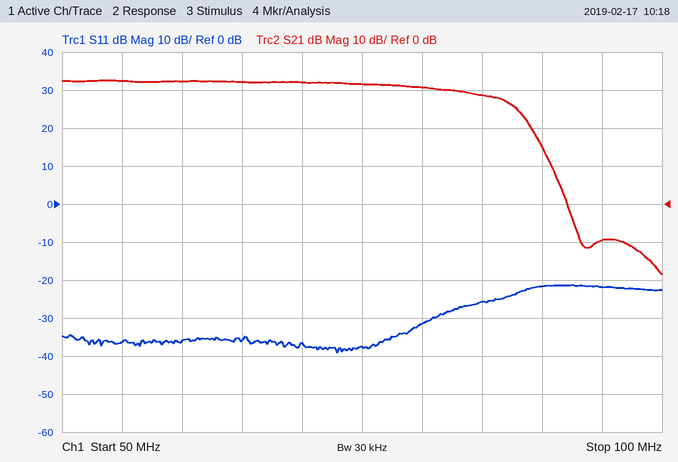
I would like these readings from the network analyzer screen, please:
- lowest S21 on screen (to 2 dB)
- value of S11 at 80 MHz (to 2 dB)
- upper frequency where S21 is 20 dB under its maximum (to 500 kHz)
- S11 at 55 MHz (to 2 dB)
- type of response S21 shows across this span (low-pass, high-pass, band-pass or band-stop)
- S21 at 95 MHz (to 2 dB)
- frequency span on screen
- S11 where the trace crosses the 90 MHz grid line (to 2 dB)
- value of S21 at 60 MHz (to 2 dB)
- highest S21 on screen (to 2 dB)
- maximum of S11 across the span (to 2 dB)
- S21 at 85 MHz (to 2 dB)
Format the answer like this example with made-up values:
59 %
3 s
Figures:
-18 dB
-32 dB
90.5 MHz
-36 dB
low-pass
-10 dB
50 MHz
-22 dB
32 dB
32 dB
-22 dB
28 dB
